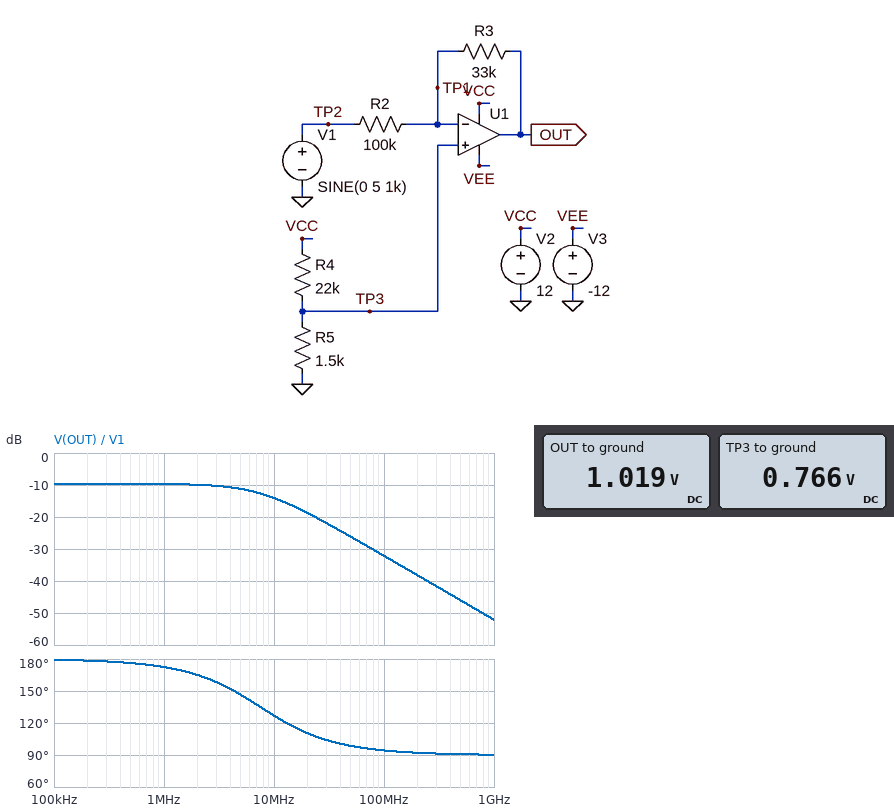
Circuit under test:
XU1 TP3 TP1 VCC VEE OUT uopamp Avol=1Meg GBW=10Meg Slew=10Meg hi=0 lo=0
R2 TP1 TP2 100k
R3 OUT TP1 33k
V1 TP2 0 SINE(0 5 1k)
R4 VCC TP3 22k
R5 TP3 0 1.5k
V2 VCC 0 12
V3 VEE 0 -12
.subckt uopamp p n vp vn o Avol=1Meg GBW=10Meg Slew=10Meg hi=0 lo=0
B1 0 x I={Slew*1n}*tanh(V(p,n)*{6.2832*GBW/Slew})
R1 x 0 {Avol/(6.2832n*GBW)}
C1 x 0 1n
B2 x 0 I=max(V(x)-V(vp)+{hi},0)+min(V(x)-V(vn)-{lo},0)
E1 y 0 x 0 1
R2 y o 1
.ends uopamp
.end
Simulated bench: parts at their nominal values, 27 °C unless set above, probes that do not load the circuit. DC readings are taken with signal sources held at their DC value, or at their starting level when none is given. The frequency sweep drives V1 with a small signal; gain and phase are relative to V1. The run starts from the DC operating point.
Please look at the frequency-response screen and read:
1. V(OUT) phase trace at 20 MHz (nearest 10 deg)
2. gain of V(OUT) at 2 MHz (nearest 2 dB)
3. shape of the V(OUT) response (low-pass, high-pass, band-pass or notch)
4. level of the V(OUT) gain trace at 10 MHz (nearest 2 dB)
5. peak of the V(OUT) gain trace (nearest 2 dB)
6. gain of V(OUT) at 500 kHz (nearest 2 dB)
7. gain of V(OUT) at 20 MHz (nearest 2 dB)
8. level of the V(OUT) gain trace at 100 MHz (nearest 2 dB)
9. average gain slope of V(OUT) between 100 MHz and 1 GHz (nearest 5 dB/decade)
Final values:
110 deg
-10 dB
low-pass
-14 dB
-10 dB
-10 dB
-18 dB
-32 dB
-20 dB/decade
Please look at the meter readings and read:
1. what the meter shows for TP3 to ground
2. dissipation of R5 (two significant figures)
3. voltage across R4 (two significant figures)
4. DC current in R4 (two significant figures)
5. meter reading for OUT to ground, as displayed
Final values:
0.766 V
390 µW
11 V
510 µA
1.019 V
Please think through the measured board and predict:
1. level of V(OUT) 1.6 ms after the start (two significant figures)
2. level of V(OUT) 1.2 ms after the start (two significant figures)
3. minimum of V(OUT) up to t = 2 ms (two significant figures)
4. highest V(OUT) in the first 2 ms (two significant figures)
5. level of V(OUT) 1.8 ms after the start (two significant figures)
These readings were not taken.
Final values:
2.0 V
-550 mV
-630 mV
2.7 V
2.6 V
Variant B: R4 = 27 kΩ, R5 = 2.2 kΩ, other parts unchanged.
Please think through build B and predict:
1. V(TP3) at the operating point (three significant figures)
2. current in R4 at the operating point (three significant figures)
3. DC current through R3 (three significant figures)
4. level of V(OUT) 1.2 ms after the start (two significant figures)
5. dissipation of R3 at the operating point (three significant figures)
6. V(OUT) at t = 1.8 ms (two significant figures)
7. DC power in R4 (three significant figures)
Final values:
904 mV
411 µA
9.04 µA
-370 mV
2.70 µW
2.8 V
4.56 mW
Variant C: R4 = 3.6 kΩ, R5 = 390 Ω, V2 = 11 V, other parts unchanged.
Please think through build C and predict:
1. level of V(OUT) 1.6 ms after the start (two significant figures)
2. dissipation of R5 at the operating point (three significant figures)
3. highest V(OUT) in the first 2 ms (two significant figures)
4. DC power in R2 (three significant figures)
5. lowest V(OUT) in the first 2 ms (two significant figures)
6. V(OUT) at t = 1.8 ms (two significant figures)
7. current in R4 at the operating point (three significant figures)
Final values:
2.4 V
2.96 mW
3.1 V
11.6 µW
-220 mV
3.0 V
2.76 mA
